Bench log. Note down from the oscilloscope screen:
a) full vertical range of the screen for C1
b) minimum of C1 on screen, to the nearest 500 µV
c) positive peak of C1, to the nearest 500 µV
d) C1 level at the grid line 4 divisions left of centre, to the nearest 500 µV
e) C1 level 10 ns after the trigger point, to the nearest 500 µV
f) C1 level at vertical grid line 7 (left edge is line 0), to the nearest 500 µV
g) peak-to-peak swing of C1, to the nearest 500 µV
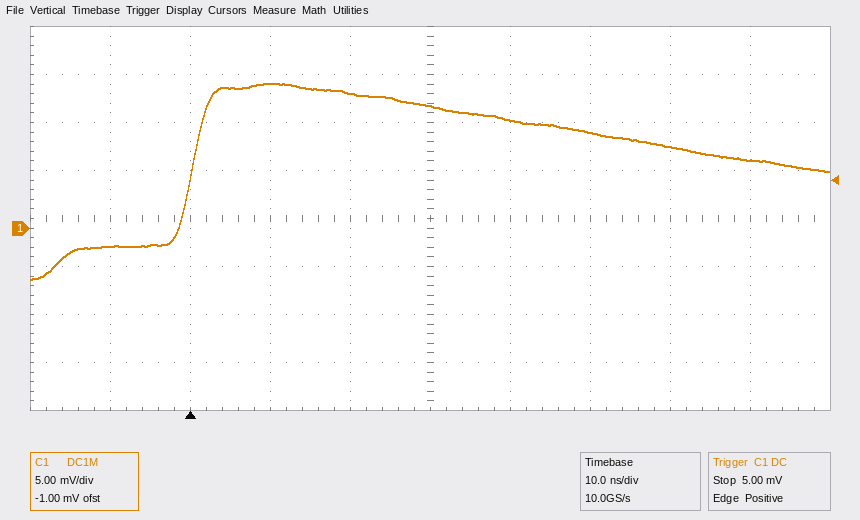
40 mV
-5.5 mV
15.0 mV
-2.0 mV
15.0 mV
10.0 mV
20.5 mV
